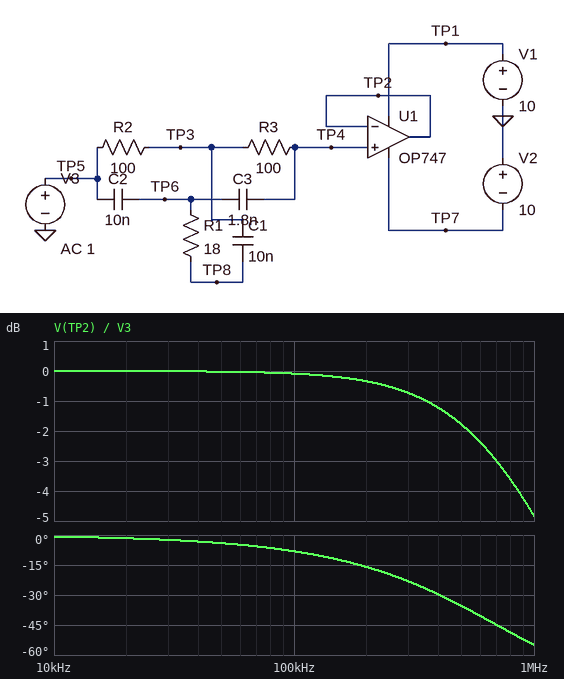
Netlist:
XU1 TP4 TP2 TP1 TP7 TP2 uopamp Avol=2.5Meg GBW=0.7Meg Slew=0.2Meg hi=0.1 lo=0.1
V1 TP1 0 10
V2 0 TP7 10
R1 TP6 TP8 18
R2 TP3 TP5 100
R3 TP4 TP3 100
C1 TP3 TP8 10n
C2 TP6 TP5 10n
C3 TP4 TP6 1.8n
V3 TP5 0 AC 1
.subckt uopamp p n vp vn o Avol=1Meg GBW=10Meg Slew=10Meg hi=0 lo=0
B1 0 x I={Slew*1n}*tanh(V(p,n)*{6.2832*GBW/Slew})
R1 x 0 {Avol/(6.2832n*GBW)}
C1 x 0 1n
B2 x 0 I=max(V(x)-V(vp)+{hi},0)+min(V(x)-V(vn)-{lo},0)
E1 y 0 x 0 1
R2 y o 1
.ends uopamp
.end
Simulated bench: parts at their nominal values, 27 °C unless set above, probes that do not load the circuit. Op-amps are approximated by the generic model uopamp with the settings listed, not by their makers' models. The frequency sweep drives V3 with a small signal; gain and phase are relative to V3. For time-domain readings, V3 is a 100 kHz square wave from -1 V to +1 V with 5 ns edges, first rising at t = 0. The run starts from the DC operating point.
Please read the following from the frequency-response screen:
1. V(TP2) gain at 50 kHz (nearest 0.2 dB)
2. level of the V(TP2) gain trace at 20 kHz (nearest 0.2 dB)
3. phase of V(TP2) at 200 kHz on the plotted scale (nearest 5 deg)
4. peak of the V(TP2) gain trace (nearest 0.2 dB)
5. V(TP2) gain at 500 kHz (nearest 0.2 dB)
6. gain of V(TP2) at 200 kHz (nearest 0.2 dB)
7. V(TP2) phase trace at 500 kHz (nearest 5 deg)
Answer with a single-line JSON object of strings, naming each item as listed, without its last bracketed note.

{"V(TP2) gain at 50 kHz": "0 dB", "level of the V(TP2) gain trace at 20 kHz": "0 dB", "phase of V(TP2) at 200 kHz on the plotted scale": "-15 deg", "peak of the V(TP2) gain trace": "0 dB", "V(TP2) gain at 500 kHz": "-1.8 dB", "gain of V(TP2) at 200 kHz": "-0.4 dB", "V(TP2) phase trace at 500 kHz": "-35 deg"}
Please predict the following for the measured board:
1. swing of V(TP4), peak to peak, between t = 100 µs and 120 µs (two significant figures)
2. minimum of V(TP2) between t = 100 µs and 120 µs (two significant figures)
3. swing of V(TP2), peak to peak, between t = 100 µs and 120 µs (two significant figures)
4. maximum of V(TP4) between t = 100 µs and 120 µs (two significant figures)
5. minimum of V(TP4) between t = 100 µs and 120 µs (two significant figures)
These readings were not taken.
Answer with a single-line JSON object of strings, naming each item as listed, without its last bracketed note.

{"swing of V(TP4), peak to peak, between t = 100 µs and 120 µs": "2.0 V", "minimum of V(TP2) between t = 100 µs and 120 µs": "-930 mV", "swing of V(TP2), peak to peak, between t = 100 µs and 120 µs": "1.0 V", "maximum of V(TP4) between t = 100 µs and 120 µs": "1.0 V", "minimum of V(TP4) between t = 100 µs and 120 µs": "-1.0 V"}
